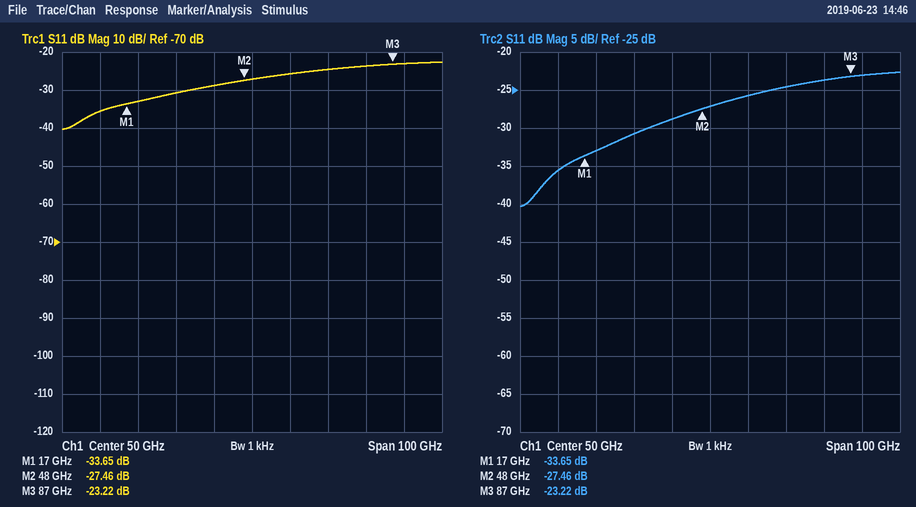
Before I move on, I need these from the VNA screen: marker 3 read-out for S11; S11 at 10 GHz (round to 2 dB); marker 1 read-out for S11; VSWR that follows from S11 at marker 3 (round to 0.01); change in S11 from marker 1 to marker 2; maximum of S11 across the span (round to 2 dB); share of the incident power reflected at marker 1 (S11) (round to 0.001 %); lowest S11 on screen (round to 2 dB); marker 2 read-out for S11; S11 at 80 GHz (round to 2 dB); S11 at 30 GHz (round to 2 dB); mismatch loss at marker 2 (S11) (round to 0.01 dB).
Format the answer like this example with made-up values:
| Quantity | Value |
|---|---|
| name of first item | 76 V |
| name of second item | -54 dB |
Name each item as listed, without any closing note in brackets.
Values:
| Quantity | Value |
|---|---|
| marker 3 read-out for S11 | -23.22 dB |
| S11 at 10 GHz | -36 dB |
| marker 1 read-out for S11 | -33.65 dB |
| VSWR that follows from S11 at marker 3 | 1.15 |
| change in S11 from marker 1 to marker 2 | 6.19 dB |
| maximum of S11 across the span | -22 dB |
| share of the incident power reflected at marker 1 (S11) | 0.043 % |
| lowest S11 on screen | -40 dB |
| marker 2 read-out for S11 | -27.46 dB |
| S11 at 80 GHz | -24 dB |
| S11 at 30 GHz | -30 dB |
| mismatch loss at marker 2 (S11) | 0.01 dB |
